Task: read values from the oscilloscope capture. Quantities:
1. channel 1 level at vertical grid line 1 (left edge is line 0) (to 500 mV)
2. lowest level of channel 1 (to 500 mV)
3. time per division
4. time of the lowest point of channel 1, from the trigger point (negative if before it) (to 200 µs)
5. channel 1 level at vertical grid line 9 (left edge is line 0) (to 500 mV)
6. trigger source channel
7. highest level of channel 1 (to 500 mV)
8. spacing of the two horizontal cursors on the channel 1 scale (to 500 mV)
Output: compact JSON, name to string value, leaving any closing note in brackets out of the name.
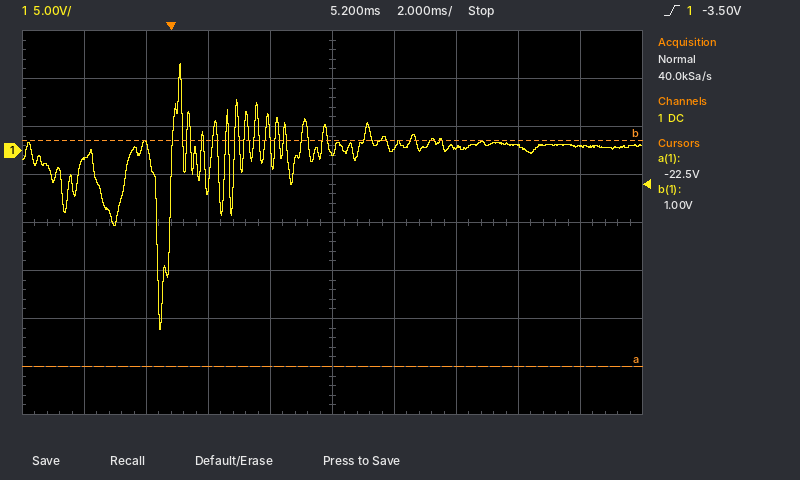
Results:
{"channel 1 level at vertical grid line 1 (left edge is line 0)": "-1.0 V", "lowest level of channel 1": "-18.5 V", "time per division": "2 ms", "time of the lowest point of channel 1, from the trigger point (negative if before it)": "-400 µs", "channel 1 level at vertical grid line 9 (left edge is line 0)": "500 mV", "trigger source channel": "channel 1", "highest level of channel 1": "9.0 V", "spacing of the two horizontal cursors on the channel 1 scale": "23.5 V"}
